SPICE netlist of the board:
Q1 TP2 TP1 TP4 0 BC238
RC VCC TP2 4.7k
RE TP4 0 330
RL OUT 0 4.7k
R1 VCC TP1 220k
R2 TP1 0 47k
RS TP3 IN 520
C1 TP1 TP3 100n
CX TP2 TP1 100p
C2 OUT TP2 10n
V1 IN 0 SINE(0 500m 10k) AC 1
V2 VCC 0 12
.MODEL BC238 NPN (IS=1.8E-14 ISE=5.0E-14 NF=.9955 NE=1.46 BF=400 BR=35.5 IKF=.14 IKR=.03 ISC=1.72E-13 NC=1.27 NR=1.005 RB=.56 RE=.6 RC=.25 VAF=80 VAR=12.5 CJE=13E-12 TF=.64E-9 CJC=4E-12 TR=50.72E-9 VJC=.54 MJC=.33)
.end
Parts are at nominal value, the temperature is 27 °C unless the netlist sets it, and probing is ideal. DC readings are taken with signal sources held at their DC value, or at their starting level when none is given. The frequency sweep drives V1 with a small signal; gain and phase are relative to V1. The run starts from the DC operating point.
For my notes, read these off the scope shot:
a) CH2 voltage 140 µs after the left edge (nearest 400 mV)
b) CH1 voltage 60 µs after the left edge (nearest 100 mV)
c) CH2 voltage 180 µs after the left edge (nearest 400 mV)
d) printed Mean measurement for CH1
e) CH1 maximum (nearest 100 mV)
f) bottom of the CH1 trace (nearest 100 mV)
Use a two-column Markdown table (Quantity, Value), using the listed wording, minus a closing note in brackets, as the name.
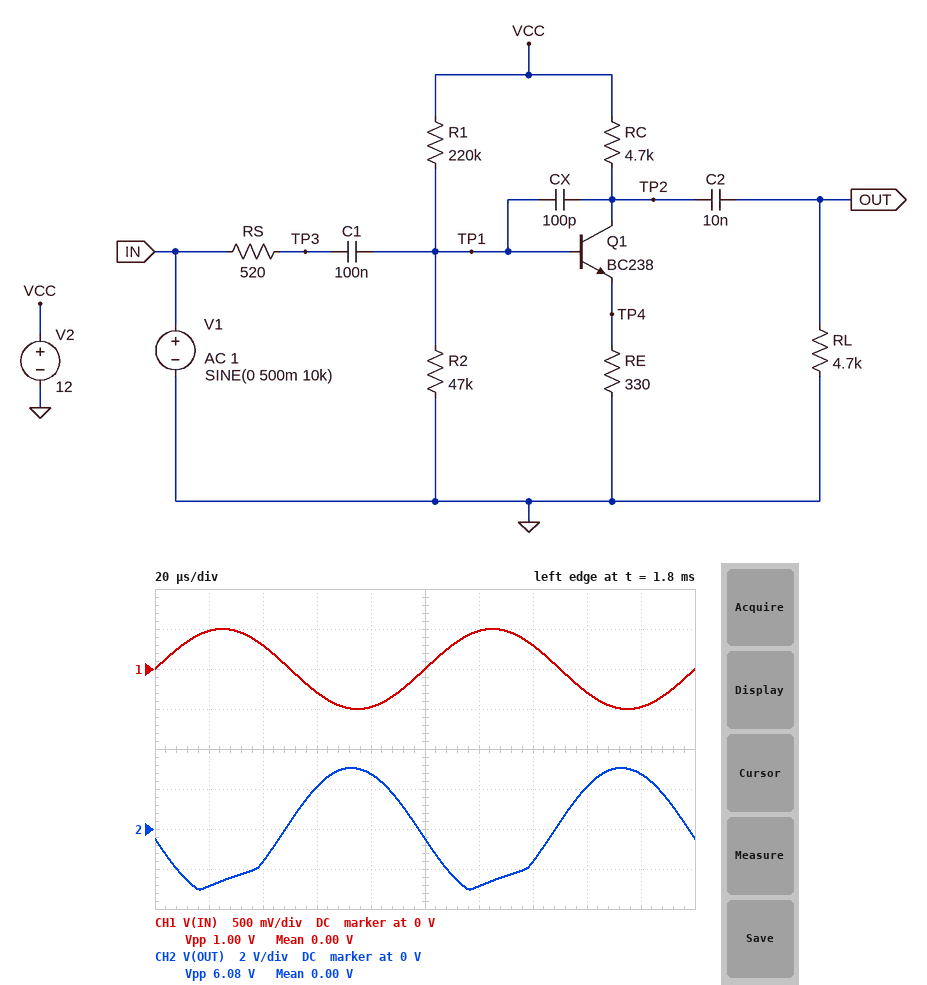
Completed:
| Quantity | Value |
|---|---|
| CH2 voltage 140 µs after the left edge | -1.6 V |
| CH1 voltage 60 µs after the left edge | -300 mV |
| CH2 voltage 180 µs after the left edge | 2.8 V |
| printed Mean measurement for CH1 | 0.00 V |
| CH1 maximum | 500 mV |
| bottom of the CH1 trace | -500 mV |
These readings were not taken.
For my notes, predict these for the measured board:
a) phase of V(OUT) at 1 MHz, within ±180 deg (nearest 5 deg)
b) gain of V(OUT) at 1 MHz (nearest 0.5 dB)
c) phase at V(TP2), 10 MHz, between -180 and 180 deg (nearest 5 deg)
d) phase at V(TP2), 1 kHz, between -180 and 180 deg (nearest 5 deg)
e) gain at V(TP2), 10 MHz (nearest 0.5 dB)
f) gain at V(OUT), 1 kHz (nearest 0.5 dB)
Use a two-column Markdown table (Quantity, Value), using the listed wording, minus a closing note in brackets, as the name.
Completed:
| Quantity | Value |
|---|---|
| phase of V(OUT) at 1 MHz, within ±180 deg | 75 deg |
| gain of V(OUT) at 1 MHz | -3.5 dB |
| phase at V(TP2), 10 MHz, between -180 and 180 deg | 10 deg |
| phase at V(TP2), 1 kHz, between -180 and 180 deg | -130 deg |
| gain at V(TP2), 10 MHz | -8.5 dB |
| gain at V(OUT), 1 kHz | -7.5 dB |
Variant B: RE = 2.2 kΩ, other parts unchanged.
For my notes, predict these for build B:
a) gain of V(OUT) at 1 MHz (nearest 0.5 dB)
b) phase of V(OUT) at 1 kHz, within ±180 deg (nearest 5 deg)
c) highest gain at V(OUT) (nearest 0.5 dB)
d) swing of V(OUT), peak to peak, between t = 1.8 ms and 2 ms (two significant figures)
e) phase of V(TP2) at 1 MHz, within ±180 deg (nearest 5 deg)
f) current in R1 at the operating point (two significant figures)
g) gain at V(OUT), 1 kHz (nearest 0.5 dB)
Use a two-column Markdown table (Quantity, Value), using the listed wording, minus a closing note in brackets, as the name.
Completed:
| Quantity | Value |
|---|---|
| gain of V(OUT) at 1 MHz | -2.5 dB |
| phase of V(OUT) at 1 kHz, within ±180 deg | -120 deg |
| highest gain at V(OUT) | 0 dB |
| swing of V(OUT), peak to peak, between t = 1.8 ms and 2 ms | 1.0 V |
| phase of V(TP2) at 1 MHz, within ±180 deg | 60 deg |
| current in R1 at the operating point | 45 µA |
| gain at V(OUT), 1 kHz | -5.5 dB |
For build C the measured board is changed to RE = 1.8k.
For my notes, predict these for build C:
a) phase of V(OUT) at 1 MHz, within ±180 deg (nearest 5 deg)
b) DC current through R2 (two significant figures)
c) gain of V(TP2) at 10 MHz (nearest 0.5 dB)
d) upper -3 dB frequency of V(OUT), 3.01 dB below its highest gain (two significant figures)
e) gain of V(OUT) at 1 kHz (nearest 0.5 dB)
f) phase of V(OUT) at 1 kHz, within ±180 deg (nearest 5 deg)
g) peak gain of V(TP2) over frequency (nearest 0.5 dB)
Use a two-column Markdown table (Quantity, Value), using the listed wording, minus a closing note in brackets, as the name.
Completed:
| Quantity | Value |
|---|---|
| phase of V(OUT) at 1 MHz, within ±180 deg | 65 deg |
| DC current through R2 | 43 µA |
| gain of V(TP2) at 10 MHz | -3.5 dB |
| upper -3 dB frequency of V(OUT), 3.01 dB below its highest gain | 680 kHz |
| gain of V(OUT) at 1 kHz | -4.0 dB |
| phase of V(OUT) at 1 kHz, within ±180 deg | -120 deg |
| peak gain of V(TP2) over frequency | 8.0 dB |
